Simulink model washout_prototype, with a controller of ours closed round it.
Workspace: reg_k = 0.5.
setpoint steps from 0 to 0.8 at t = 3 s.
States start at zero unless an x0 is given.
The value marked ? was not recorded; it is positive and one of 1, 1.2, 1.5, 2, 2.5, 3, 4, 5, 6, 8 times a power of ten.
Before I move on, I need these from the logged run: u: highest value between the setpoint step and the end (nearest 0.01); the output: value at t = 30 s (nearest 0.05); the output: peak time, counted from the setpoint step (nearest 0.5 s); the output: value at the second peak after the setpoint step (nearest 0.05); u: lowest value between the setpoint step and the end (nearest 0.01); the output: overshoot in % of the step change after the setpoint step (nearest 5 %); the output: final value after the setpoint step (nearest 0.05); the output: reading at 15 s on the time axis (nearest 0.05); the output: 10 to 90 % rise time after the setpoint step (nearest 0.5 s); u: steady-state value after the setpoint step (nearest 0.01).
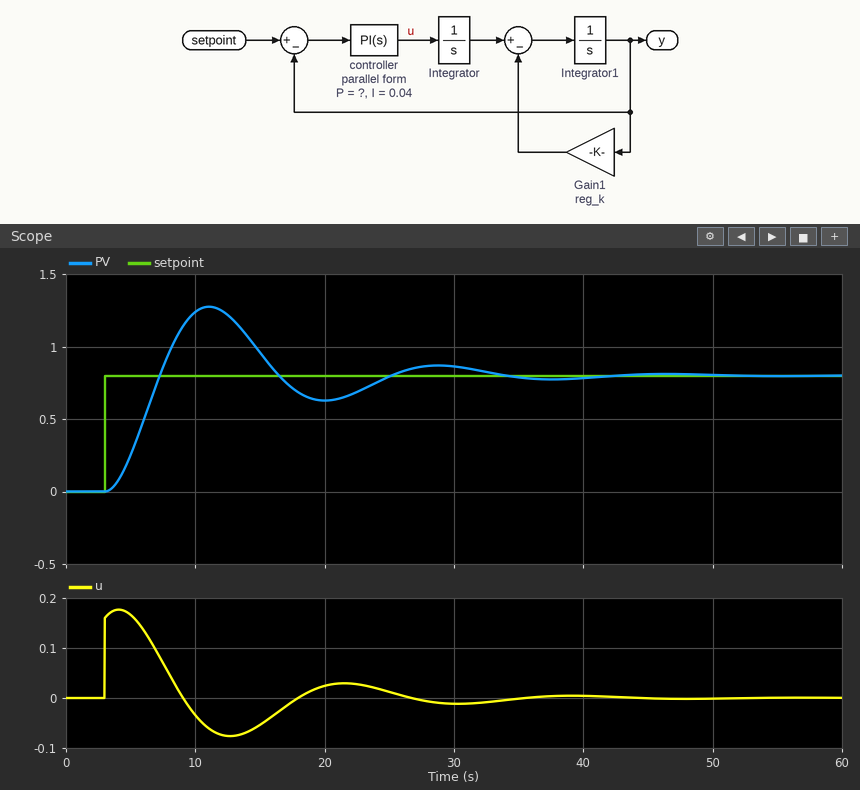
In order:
0.18
0.85
8.0 s
0.85
-0.08
60 %
0.80
0.95
3.0 s
0.00
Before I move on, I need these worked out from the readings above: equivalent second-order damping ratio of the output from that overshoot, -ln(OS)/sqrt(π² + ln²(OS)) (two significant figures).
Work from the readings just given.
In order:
0.16
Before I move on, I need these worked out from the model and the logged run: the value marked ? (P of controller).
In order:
0.2
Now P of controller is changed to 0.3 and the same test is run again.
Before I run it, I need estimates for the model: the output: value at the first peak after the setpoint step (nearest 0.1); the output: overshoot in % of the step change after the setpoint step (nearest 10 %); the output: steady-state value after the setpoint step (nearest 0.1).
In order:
1.2
50 %
0.8
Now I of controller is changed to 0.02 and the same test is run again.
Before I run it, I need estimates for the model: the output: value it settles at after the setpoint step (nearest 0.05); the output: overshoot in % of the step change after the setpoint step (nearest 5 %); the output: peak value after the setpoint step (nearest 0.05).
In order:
0.80
40 %
1.10
